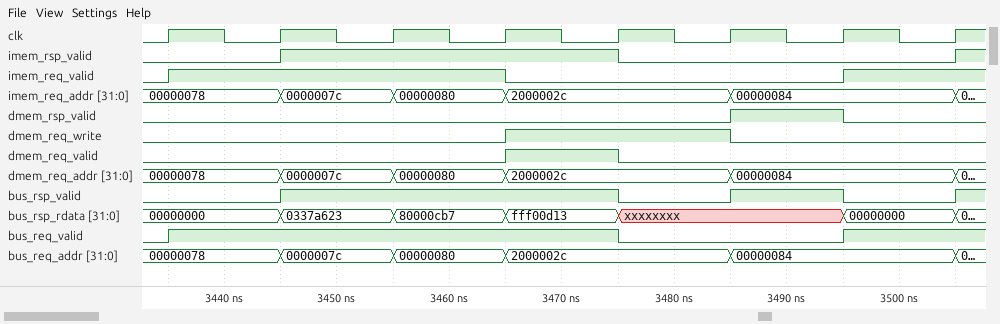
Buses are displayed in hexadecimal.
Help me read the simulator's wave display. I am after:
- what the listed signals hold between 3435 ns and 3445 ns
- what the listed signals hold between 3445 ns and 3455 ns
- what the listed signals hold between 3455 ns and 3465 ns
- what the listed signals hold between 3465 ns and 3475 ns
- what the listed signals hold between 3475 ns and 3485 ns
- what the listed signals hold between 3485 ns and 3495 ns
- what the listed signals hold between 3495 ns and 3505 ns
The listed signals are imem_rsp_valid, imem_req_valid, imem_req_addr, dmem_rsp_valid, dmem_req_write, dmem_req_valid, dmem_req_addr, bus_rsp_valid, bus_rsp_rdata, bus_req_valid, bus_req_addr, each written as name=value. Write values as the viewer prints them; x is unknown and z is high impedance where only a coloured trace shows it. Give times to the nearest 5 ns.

imem_rsp_valid=0, imem_req_valid=1, imem_req_addr=00000078, dmem_rsp_valid=0, dmem_req_write=0, dmem_req_valid=0, dmem_req_addr=00000078, bus_rsp_valid=0, bus_rsp_rdata=00000000, bus_req_valid=1, bus_req_addr=00000078
imem_rsp_valid=1, imem_req_valid=1, imem_req_addr=0000007c, dmem_rsp_valid=0, dmem_req_write=0, dmem_req_valid=0, dmem_req_addr=0000007c, bus_rsp_valid=1, bus_rsp_rdata=0337a623, bus_req_valid=1, bus_req_addr=0000007c
imem_rsp_valid=1, imem_req_valid=1, imem_req_addr=00000080, dmem_rsp_valid=0, dmem_req_write=0, dmem_req_valid=0, dmem_req_addr=00000080, bus_rsp_valid=1, bus_rsp_rdata=80000cb7, bus_req_valid=1, bus_req_addr=00000080
imem_rsp_valid=1, imem_req_valid=0, imem_req_addr=2000002c, dmem_rsp_valid=0, dmem_req_write=1, dmem_req_valid=1, dmem_req_addr=2000002c, bus_rsp_valid=1, bus_rsp_rdata=fff00d13, bus_req_valid=1, bus_req_addr=2000002c
imem_rsp_valid=0, imem_req_valid=0, imem_req_addr=2000002c, dmem_rsp_valid=0, dmem_req_write=1, dmem_req_valid=0, dmem_req_addr=2000002c, bus_rsp_valid=0, bus_rsp_rdata=xxxxxxxx, bus_req_valid=0, bus_req_addr=2000002c
imem_rsp_valid=0, imem_req_valid=0, imem_req_addr=00000084, dmem_rsp_valid=1, dmem_req_write=0, dmem_req_valid=0, dmem_req_addr=00000084, bus_rsp_valid=1, bus_rsp_rdata=xxxxxxxx, bus_req_valid=0, bus_req_addr=00000084
imem_rsp_valid=0, imem_req_valid=1, imem_req_addr=00000084, dmem_rsp_valid=0, dmem_req_write=0, dmem_req_valid=0, dmem_req_addr=00000084, bus_rsp_valid=0, bus_rsp_rdata=00000000, bus_req_valid=1, bus_req_addr=00000084
